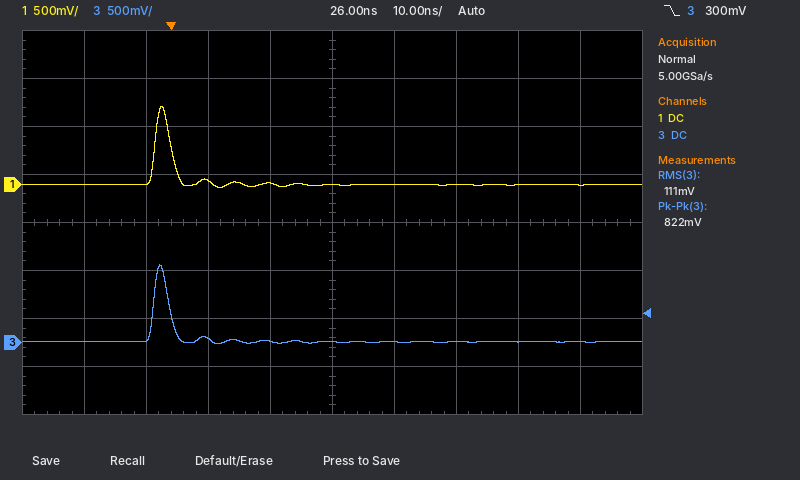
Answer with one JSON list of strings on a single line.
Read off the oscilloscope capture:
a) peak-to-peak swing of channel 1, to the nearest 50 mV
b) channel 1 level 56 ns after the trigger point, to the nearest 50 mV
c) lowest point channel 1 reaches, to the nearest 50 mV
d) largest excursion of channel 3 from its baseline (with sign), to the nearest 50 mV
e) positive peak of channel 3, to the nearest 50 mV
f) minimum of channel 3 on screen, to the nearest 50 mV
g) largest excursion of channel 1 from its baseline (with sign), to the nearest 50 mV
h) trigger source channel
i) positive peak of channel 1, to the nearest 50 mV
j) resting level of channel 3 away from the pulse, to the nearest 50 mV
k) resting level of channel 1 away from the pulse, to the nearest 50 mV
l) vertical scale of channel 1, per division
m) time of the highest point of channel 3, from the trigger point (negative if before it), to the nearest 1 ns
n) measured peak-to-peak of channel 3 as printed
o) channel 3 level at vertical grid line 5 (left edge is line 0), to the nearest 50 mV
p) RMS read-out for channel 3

["850 mV", "0 mV", "-50 mV", "+800 mV", "800 mV", "0 mV", "+800 mV", "channel 3", "800 mV", "0 mV", "0 mV", "500 mV", "-2 ns", "822 mV", "0 mV", "111 mV"]
